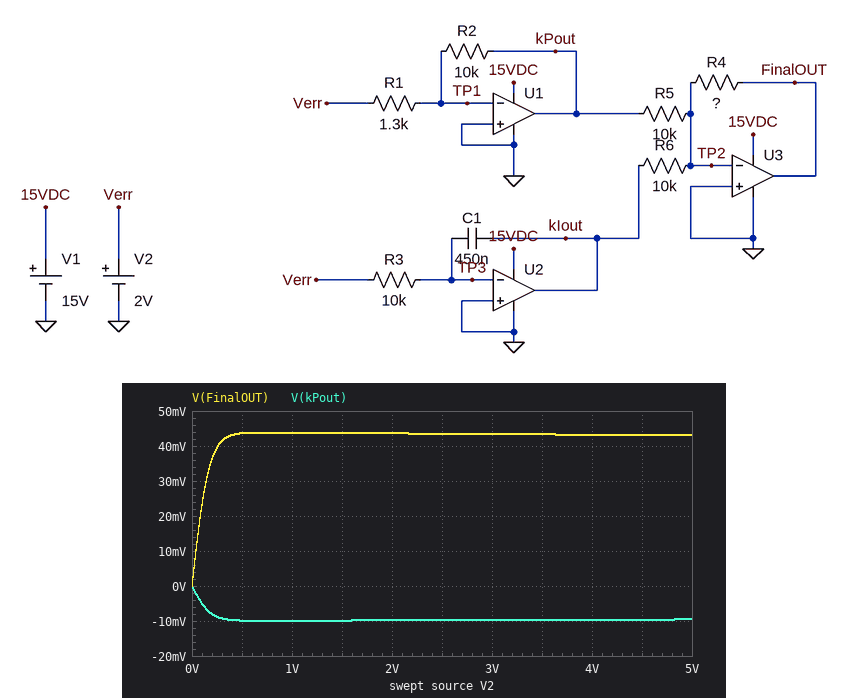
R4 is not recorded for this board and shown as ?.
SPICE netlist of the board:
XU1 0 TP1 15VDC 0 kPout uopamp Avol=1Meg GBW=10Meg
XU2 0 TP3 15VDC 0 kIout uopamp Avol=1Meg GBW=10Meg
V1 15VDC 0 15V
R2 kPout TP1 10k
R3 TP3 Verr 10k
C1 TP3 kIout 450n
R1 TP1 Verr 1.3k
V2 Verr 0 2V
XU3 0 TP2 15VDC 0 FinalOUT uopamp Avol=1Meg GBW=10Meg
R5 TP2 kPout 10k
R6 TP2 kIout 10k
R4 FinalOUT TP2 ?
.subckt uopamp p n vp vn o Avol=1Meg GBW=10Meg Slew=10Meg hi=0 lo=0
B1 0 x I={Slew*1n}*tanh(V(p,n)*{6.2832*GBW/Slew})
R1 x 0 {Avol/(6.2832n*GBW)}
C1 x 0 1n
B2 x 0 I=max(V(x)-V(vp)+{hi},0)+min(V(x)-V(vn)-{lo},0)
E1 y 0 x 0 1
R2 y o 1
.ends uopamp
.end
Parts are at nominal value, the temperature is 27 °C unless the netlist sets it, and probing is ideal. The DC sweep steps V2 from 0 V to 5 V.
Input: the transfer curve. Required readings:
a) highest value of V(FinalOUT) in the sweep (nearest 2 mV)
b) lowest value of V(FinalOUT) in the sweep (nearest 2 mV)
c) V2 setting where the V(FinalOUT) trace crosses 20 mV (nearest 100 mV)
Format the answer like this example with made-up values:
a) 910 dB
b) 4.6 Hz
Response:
a) 44 mV
b) 0 V
c) 100 mV
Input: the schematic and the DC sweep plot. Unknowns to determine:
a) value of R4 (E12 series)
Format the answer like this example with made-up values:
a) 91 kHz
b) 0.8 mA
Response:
a) 22 kΩ
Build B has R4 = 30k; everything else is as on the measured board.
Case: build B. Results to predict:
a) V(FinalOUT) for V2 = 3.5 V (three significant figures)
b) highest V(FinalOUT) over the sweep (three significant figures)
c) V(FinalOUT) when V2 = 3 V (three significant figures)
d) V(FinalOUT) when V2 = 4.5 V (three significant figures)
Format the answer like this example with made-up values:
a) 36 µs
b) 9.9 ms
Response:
a) 59.1 mV
b) 59.8 mV
c) 59.2 mV
d) 58.8 mV
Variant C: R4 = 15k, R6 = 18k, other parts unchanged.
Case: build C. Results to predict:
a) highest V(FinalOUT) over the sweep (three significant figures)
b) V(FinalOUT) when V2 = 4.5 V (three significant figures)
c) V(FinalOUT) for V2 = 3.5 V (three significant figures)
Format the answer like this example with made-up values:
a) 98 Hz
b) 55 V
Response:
a) 23.2 mV
b) 22.7 mV
c) 22.9 mV
